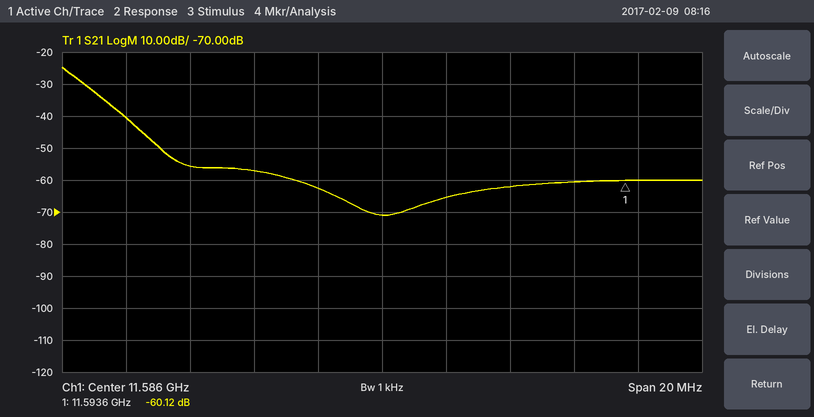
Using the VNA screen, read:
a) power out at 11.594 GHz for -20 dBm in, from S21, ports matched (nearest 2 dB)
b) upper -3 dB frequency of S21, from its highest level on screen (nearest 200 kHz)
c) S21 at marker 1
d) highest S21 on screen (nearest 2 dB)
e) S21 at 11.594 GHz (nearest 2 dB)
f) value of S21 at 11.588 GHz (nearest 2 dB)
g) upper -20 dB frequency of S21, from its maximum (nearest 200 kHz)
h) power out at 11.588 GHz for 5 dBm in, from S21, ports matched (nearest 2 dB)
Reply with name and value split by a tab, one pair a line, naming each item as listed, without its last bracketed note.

power out at 11.594 GHz for -20 dBm in, from S21, ports matched	-80 dBm
upper -3 dB frequency of S21, from its highest level on screen	11.5764 GHz
S21 at marker 1	-60.12 dB
highest S21 on screen	-24 dB
S21 at 11.594 GHz	-60 dB
value of S21 at 11.588 GHz	-66 dB
upper -20 dB frequency of S21, from its maximum	11.5784 GHz
power out at 11.588 GHz for 5 dBm in, from S21, ports matched	-60 dBm
